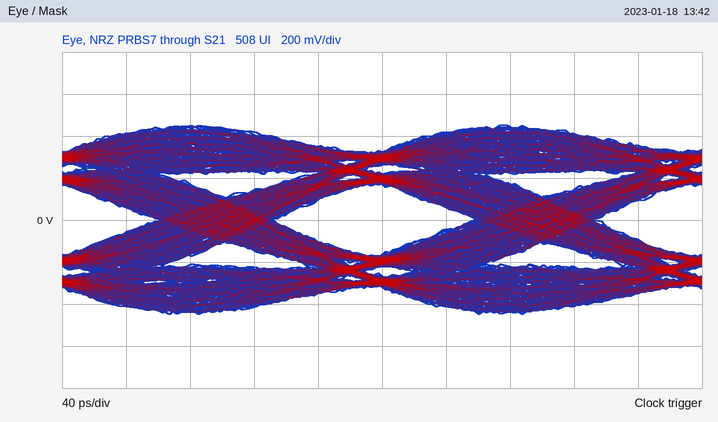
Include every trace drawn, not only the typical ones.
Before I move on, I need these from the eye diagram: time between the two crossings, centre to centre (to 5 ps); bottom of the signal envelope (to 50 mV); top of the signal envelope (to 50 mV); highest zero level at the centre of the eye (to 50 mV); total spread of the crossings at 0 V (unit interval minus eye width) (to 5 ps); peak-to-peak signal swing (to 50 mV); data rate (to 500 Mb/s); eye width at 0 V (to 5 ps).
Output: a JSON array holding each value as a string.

["200 ps", "-450 mV", "450 mV", "-150 mV", "75 ps", "900 mV", "5.0 Gb/s", "125 ps"]
